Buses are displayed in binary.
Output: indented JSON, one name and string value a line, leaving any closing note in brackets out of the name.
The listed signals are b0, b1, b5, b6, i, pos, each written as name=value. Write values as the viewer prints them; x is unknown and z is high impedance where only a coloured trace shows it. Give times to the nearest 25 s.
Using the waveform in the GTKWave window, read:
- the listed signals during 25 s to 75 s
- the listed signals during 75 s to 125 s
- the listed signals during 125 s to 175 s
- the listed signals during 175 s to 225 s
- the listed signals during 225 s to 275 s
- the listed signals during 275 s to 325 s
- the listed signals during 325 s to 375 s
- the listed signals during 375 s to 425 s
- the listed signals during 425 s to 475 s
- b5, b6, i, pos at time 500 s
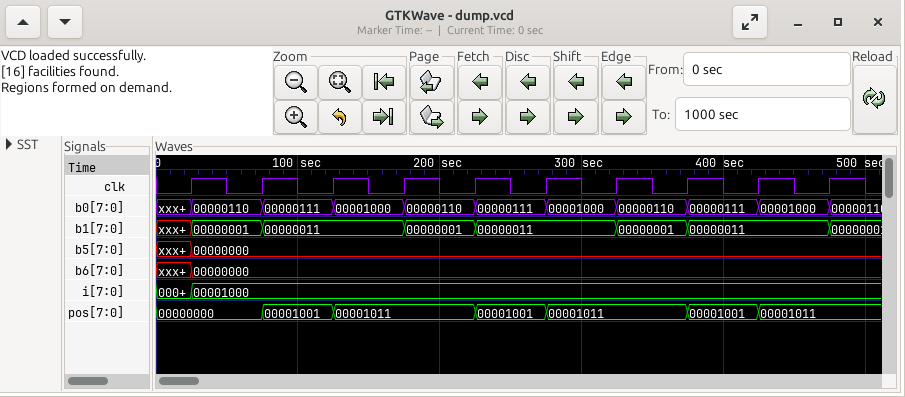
{
  "the listed signals during 25 s to 75 s": "b0=00000110, b1=00000001, b5=00000000, b6=00000000, i=00001000, pos=00000000",
  "the listed signals during 75 s to 125 s": "b0=00000111, b1=00000011, b5=00000000, b6=00000000, i=00001000, pos=00001001",
  "the listed signals during 125 s to 175 s": "b0=00001000, b1=00000011, b5=00000000, b6=00000000, i=00001000, pos=00001011",
  "the listed signals during 175 s to 225 s": "b0=00000110, b1=00000001, b5=00000000, b6=00000000, i=00001000, pos=00001011",
  "the listed signals during 225 s to 275 s": "b0=00000111, b1=00000011, b5=00000000, b6=00000000, i=00001000, pos=00001001",
  "the listed signals during 275 s to 325 s": "b0=00001000, b1=00000011, b5=00000000, b6=00000000, i=00001000, pos=00001011",
  "the listed signals during 325 s to 375 s": "b0=00000110, b1=00000001, b5=00000000, b6=00000000, i=00001000, pos=00001011",
  "the listed signals during 375 s to 425 s": "b0=00000111, b1=00000011, b5=00000000, b6=00000000, i=00001000, pos=00001001",
  "the listed signals during 425 s to 475 s": "b0=00001000, b1=00000011, b5=00000000, b6=00000000, i=00001000, pos=00001011",
  "b5, b6, i, pos at time 500 s": "b5=00000000, b6=00000000, i=00001000, pos=00001011"
}
